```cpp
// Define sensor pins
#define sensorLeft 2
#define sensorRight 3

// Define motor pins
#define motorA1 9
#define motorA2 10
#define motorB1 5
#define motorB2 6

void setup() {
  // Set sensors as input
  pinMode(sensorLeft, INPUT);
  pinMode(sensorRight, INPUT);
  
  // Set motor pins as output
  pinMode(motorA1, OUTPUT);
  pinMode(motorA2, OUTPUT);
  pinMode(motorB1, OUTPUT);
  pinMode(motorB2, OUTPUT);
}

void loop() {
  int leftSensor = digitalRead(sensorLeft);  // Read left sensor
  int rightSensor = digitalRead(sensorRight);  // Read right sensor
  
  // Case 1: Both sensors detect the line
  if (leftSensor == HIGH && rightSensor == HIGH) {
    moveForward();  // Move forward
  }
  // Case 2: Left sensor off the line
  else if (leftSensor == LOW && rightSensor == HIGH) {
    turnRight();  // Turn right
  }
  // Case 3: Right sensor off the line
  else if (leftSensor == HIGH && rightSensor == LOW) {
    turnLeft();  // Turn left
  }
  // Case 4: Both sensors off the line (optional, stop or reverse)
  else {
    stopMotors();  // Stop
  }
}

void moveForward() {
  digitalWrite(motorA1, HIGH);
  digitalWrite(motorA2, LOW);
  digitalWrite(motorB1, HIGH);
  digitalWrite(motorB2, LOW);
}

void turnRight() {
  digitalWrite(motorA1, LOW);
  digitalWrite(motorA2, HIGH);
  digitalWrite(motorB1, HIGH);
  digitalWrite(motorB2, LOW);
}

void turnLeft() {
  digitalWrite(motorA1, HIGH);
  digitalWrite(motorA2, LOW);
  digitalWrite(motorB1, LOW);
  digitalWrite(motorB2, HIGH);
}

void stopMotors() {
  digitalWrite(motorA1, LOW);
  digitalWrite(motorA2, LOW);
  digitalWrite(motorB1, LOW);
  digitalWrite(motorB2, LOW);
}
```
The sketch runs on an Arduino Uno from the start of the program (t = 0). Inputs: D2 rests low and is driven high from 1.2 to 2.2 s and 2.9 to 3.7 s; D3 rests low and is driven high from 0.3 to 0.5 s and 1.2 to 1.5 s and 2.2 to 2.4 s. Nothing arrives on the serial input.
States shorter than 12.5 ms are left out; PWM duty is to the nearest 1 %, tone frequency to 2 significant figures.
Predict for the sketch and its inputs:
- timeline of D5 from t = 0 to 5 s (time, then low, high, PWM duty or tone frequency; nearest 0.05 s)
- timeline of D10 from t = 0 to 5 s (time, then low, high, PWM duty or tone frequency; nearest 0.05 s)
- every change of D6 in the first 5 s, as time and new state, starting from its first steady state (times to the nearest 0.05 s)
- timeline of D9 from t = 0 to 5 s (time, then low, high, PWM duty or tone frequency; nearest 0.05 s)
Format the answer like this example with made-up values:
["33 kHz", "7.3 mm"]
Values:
["0 s low; 0.3 s high; 0.5 s low; 1.2 s high; 1.5 s low; 2.2 s high; 2.4 s low", "0 s low; 0.3 s high; 0.5 s low; 2.2 s high; 2.4 s low", "0 s low; 1.5 s high; 2.2 s low; 2.9 s high; 3.7 s low", "0 s low; 1.2 s high; 2.2 s low; 2.9 s high; 3.7 s low"]
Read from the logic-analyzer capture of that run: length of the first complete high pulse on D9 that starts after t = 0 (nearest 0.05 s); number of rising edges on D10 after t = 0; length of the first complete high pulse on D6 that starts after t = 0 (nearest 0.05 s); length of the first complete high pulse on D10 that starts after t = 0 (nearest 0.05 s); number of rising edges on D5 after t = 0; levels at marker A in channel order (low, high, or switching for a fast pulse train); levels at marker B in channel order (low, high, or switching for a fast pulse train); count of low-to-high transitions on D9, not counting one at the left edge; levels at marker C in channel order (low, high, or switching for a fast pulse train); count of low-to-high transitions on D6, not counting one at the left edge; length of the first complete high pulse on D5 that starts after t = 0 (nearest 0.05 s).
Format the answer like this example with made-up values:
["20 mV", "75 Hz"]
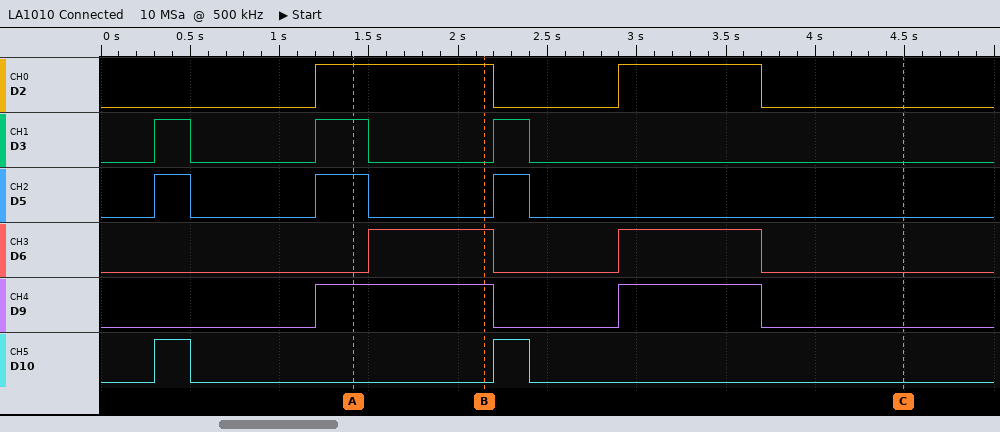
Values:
["1.00 s", "2", "0.70 s", "0.20 s", "3", "D2 high, D3 high, D5 high, D6 low, D9 high, D10 low", "D2 high, D3 low, D5 low, D6 high, D9 high, D10 low", "2", "D2 low, D3 low, D5 low, D6 low, D9 low, D10 low", "2", "0.20 s"]
